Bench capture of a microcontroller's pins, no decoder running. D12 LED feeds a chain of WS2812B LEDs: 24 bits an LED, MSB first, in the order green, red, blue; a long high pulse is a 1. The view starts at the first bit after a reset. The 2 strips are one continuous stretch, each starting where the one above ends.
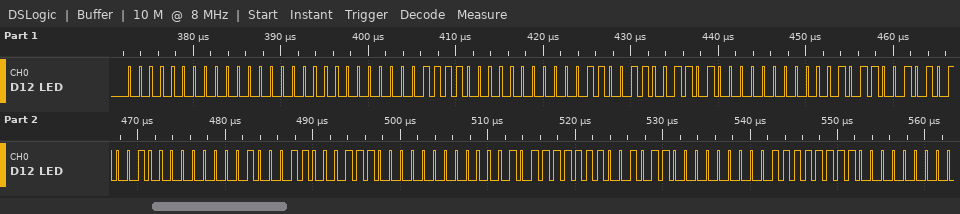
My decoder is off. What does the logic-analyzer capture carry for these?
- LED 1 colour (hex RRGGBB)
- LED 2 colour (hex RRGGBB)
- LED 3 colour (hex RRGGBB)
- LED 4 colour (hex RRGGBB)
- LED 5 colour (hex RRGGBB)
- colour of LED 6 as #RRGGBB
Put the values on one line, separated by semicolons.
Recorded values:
#000000; #001E33; #003459; #00528C; #0070BF; #0096FF
